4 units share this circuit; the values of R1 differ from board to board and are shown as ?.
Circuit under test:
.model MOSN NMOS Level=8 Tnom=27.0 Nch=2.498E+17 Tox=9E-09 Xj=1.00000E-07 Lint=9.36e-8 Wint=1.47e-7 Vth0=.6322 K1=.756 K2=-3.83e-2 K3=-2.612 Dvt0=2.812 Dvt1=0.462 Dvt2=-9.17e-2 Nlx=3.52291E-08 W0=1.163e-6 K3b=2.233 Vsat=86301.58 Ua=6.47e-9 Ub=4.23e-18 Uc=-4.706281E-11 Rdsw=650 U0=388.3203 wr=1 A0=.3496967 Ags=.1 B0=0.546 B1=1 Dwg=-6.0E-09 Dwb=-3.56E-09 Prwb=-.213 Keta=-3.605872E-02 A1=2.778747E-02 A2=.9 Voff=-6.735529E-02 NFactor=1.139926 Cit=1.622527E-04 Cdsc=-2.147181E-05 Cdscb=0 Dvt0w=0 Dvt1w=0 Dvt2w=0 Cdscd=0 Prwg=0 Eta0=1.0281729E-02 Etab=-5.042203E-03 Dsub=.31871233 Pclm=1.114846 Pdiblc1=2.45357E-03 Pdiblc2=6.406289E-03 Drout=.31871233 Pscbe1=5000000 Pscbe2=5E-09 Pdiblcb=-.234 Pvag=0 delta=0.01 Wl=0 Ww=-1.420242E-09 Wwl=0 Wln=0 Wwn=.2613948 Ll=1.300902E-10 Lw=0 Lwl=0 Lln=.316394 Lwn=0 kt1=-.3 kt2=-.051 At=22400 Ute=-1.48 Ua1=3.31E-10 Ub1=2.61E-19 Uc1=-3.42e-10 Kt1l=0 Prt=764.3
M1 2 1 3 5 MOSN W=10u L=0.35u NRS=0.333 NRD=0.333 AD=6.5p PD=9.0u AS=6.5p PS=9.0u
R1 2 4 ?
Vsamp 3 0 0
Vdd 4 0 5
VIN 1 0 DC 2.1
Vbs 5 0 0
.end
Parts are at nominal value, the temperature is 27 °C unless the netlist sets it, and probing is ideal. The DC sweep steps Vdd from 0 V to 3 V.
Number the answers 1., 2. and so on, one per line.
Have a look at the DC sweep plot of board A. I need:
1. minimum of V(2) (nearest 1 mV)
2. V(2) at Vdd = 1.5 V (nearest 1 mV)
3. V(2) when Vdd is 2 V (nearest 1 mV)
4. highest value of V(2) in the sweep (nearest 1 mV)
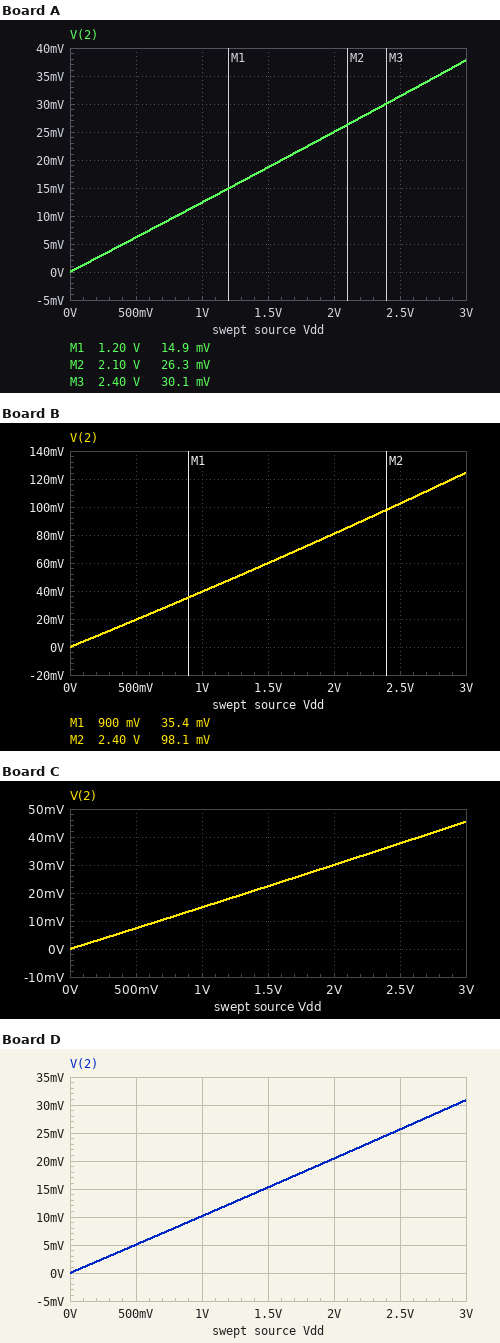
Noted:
1. 0 V
2. 19 mV
3. 25 mV
4. 38 mV
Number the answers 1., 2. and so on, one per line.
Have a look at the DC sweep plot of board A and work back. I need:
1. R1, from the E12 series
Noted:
1. 18 kΩ
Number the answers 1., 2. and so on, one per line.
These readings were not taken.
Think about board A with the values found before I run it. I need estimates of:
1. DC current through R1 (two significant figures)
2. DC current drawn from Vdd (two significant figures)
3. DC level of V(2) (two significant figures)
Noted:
1. 270 µA
2. 270 µA
3. 64 mV
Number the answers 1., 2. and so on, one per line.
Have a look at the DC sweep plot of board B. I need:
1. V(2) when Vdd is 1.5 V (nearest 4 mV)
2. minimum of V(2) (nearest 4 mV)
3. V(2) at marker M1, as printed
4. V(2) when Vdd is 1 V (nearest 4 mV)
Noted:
1. 60 mV
2. 0 V
3. 35.4 mV
4. 40 mV
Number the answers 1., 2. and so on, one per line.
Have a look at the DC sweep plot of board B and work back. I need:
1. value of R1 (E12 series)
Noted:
1. 5.6 kΩ
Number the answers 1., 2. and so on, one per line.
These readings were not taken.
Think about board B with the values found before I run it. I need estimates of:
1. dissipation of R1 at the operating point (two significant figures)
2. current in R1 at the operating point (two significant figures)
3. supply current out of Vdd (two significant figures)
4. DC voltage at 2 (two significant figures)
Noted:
1. 4.1 mW
2. 850 µA
3. 850 µA
4. 220 mV
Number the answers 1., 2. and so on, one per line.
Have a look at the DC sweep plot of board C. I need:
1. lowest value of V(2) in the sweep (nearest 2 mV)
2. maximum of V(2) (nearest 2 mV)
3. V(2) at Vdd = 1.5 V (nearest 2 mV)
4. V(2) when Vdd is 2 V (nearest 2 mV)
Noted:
1. 0 V
2. 46 mV
3. 22 mV
4. 30 mV
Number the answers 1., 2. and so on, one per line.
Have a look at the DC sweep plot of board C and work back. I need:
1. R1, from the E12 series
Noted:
1. 15 kΩ
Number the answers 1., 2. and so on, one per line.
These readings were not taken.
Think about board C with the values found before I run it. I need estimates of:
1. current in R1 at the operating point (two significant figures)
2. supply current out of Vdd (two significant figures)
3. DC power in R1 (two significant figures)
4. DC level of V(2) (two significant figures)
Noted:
1. 330 µA
2. 330 µA
3. 1.6 mW
4. 77 mV
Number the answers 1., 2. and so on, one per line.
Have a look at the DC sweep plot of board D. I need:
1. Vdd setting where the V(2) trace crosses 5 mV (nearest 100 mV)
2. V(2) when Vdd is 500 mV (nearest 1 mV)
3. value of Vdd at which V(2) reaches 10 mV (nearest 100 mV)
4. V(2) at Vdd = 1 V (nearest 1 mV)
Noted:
1. 500 mV
2. 5 mV
3. 1.0 V
4. 10 mV
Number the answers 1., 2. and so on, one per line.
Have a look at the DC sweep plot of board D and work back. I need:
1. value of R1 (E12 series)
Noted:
1. 22 kΩ
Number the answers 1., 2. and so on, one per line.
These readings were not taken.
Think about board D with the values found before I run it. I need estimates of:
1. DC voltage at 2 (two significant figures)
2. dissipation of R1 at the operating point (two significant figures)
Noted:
1. 52 mV
2. 1.1 mW
